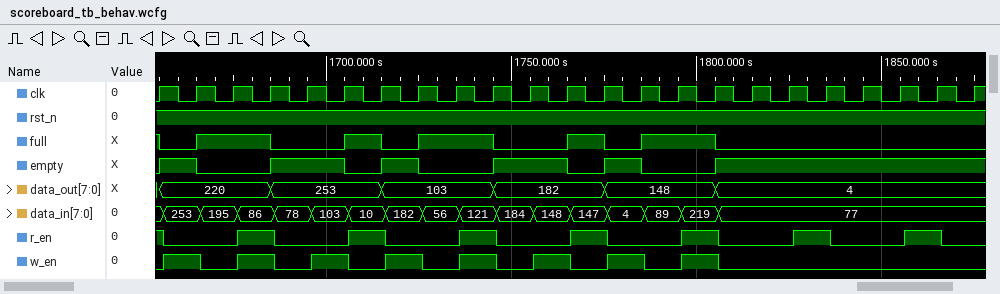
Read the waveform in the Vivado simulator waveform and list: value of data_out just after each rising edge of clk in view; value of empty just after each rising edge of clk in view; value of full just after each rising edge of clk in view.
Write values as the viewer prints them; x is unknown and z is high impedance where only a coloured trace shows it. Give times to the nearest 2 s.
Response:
220, 220, 220, 253, 253, 253, 103, 103, 103, 182, 182, 182, 148, 148, 148, 4, 4, 4, 4, 4, 4, 4, 4
1 0 0 1 1 0 1 0 0 1 1 0 1 0 0 1 1 1 1 1 1 1 1
0 1 1 0 0 1 0 1 1 0 0 1 0 1 1 0 0 0 0 0 0 0 0
